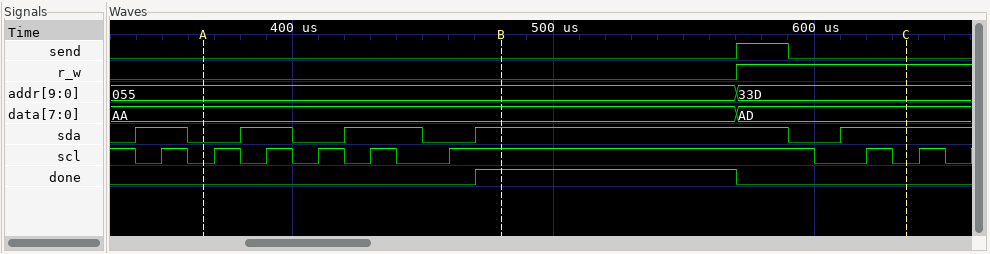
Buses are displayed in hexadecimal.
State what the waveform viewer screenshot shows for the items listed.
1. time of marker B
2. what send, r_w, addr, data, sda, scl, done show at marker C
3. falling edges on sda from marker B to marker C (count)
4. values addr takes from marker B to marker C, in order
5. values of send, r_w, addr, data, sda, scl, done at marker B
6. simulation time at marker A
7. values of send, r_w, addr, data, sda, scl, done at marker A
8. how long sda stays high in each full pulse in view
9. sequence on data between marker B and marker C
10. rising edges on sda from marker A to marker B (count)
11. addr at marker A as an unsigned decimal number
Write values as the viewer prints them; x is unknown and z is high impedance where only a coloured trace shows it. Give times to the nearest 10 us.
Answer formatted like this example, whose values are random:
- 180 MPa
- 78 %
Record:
- 480 us
- send=0, r_w=1, addr=33D, data=AD, sda=1, scl=0, done=0
- 1
- 055, 33D
- send=0, r_w=0, addr=055, data=AA, sda=1, scl=1, done=1
- 370 us
- send=0, r_w=0, addr=055, data=AA, sda=0, scl=0, done=0
- 20 us, 20 us, 30 us, 120 us
- AA, AD
- 3
- 85
